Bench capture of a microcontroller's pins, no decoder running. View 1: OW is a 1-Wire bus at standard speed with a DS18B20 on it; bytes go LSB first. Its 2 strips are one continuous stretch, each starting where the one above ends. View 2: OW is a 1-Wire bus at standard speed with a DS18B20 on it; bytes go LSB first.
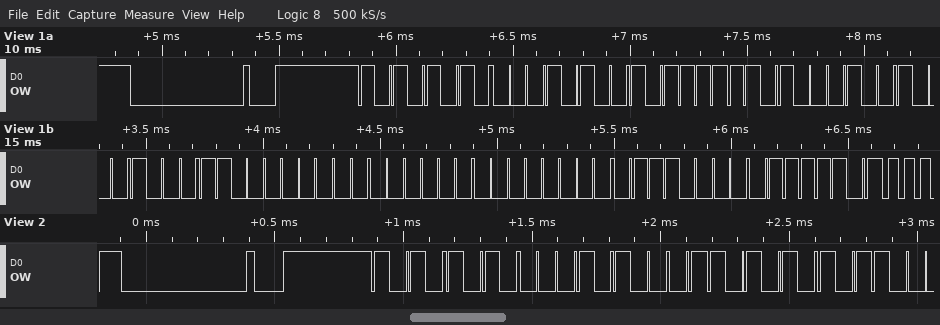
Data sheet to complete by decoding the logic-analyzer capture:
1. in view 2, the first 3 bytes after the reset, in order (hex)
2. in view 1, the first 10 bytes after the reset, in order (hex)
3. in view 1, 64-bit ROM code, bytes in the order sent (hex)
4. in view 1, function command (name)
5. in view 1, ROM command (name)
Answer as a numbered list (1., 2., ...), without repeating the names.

1. 55 28 56
2. 55 28 FD 22 11 03 00 00 0E BE
3. 28 FD 22 11 03 00 00 0E
4. Read Scratchpad
5. Match ROM
